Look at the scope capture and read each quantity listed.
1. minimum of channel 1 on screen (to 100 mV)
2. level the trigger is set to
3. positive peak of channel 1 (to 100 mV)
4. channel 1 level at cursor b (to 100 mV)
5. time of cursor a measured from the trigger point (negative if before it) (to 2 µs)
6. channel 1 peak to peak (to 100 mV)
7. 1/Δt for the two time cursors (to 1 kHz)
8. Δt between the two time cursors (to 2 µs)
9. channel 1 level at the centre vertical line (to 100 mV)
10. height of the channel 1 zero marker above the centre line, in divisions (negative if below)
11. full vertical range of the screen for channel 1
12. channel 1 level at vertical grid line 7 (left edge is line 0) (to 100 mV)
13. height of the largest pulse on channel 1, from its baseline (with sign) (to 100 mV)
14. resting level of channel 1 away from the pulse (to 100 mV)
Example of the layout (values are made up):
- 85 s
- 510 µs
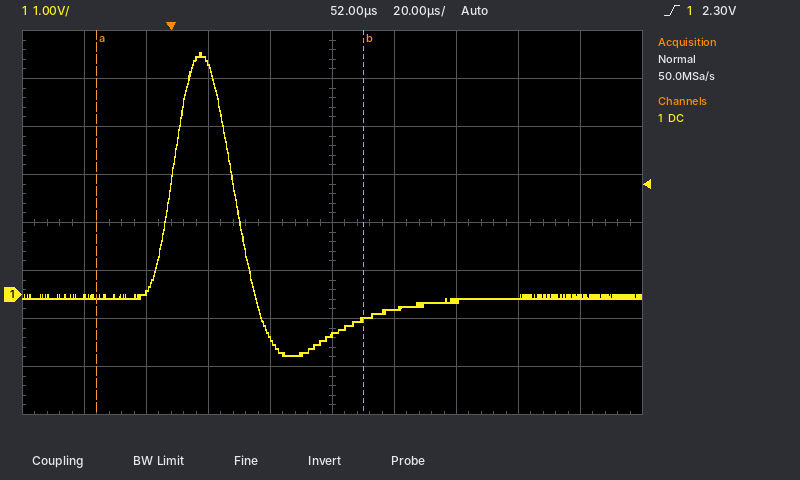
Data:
- -1.3 V
- 2.30 V
- 5.0 V
- -500 mV
- -24 µs
- 6.3 V
- 12 kHz
- 86 µs
- -800 mV
- -1.5 div
- 8 V
- -100 mV
- +5.1 V
- -100 mV
